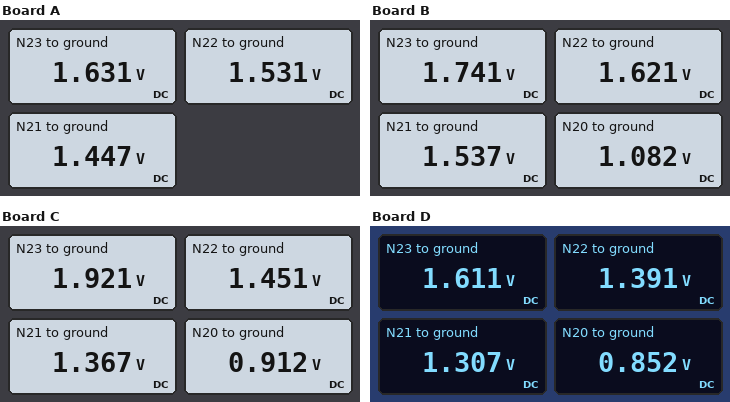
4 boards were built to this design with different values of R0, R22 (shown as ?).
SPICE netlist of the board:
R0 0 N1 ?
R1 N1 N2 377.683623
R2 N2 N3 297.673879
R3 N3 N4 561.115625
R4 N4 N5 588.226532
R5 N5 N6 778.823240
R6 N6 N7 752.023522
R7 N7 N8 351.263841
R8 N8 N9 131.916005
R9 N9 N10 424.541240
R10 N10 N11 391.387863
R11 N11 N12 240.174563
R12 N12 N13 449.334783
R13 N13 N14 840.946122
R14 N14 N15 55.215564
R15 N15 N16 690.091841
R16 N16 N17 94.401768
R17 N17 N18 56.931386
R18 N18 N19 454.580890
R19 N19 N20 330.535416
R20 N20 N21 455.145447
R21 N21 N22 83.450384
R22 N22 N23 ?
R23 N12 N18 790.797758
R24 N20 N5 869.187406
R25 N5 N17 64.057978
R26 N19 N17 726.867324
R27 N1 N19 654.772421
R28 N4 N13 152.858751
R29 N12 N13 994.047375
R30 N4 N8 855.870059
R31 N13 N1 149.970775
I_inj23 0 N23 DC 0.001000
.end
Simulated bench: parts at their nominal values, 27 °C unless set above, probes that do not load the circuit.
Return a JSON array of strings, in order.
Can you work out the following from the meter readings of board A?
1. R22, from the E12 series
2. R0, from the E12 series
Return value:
["100 Ω", "470 Ω"]
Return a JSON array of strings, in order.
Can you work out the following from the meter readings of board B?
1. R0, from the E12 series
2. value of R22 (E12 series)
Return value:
["560 Ω", "120 Ω"]
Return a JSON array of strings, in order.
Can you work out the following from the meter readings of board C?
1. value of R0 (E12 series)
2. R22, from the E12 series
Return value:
["390 Ω", "470 Ω"]
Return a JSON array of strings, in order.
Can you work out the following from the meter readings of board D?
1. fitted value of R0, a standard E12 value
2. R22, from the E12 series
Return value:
["330 Ω", "220 Ω"]
